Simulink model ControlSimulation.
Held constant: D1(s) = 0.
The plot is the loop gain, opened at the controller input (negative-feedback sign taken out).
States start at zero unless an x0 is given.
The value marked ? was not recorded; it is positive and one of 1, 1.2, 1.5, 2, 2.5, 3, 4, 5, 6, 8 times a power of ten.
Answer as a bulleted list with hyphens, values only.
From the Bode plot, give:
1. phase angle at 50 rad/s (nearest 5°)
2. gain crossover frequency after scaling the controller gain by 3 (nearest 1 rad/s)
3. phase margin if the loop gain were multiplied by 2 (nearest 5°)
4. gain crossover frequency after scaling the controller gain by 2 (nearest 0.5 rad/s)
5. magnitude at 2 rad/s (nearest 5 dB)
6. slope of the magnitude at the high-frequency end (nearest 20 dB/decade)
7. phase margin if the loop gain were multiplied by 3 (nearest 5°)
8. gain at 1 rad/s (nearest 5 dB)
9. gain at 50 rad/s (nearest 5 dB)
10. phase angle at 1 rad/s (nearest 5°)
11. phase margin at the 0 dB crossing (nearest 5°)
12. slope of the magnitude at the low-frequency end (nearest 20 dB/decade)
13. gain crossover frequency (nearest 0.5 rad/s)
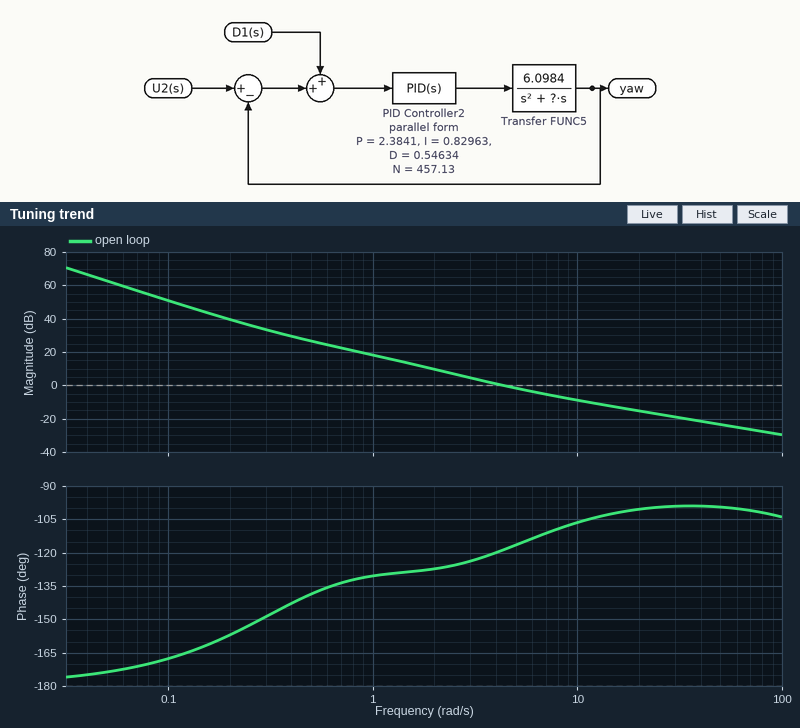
- -100°
- 11 rad/s
- 70°
- 7.5 rad/s
- 10 dB
- -20 dB/decade
- 75°
- 20 dB
- -25 dB
- -130°
- 60°
- -40 dB/decade
- 4.5 rad/s
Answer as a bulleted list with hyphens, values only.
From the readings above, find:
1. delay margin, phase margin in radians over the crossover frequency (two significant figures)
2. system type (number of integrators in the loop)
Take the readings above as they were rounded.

- 0.23 s
- 2
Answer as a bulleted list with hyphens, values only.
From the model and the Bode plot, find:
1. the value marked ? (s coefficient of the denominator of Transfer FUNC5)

- 1.5
